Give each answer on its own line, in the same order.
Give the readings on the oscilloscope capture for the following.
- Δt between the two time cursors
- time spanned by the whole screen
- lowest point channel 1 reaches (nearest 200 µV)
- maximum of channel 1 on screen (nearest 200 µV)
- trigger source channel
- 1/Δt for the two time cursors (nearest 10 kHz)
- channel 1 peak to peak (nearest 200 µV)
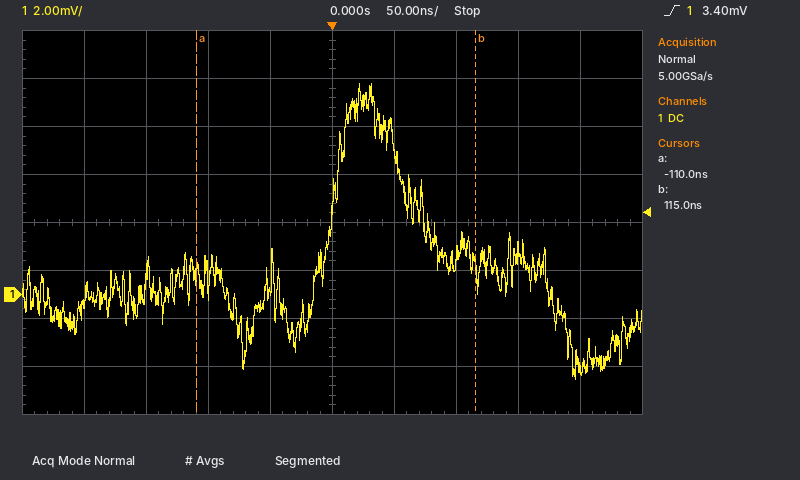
225 ns
500 ns
-3.6 mV
8.8 mV
channel 1
4.44 MHz
12.4 mV
